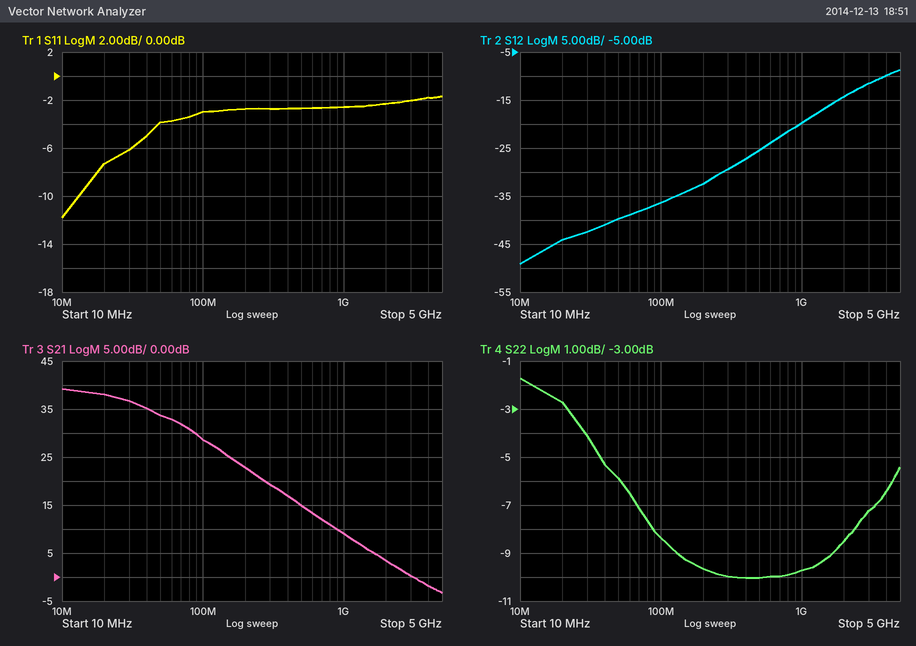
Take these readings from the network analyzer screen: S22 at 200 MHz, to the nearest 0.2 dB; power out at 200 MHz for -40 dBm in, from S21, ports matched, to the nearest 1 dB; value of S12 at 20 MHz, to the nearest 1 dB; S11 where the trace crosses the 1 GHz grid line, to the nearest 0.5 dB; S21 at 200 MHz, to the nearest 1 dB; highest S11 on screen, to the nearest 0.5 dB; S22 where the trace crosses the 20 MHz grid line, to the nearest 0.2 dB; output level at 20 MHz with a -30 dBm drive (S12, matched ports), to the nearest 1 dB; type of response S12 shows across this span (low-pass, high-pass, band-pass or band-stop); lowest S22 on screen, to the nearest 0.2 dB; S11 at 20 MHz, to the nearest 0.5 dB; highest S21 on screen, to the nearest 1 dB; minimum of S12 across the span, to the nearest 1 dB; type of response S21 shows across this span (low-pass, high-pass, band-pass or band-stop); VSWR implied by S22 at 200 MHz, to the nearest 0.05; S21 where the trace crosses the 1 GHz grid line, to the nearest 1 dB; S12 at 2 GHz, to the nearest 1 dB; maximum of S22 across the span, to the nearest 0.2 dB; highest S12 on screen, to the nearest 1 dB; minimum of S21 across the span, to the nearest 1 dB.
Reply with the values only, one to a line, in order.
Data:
-9.6 dB
-17 dBm
-44 dB
-2.5 dB
23 dB
-1.5 dB
-2.8 dB
-74 dBm
high-pass
-10.0 dB
-7.5 dB
39 dB
-49 dB
low-pass
2.00
9 dB
-14 dB
-1.8 dB
-9 dB
-3 dB
